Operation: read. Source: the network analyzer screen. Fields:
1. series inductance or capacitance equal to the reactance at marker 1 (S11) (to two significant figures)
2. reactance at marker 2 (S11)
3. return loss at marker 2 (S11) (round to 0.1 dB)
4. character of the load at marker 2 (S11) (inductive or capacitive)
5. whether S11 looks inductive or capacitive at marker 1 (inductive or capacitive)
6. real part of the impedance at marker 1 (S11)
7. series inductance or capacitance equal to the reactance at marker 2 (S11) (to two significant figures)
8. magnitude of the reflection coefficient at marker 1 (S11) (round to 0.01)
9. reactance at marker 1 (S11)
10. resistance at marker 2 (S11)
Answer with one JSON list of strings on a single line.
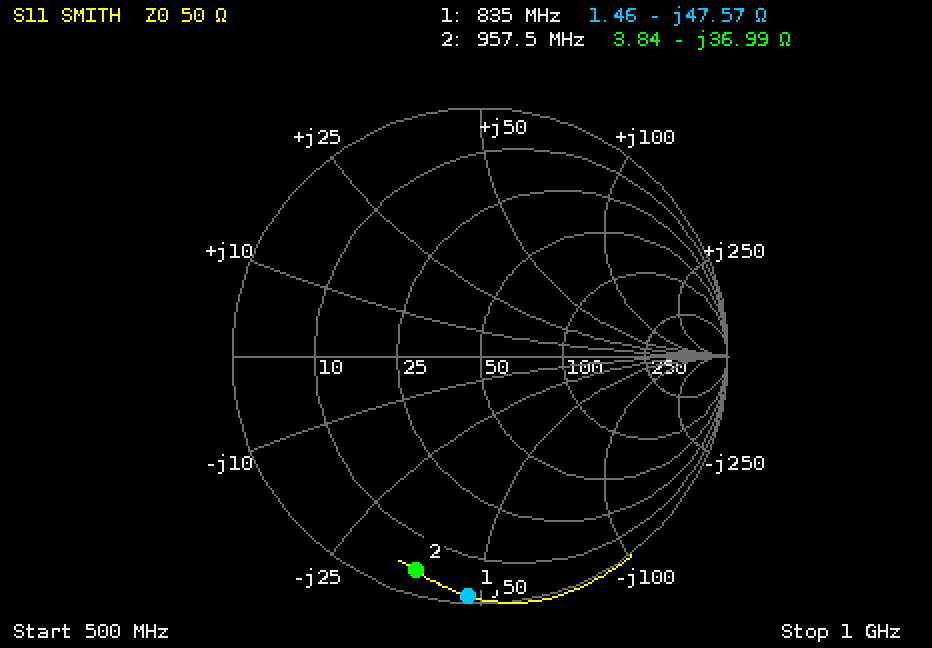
["4.0 pF", "-36.99 Ω", "0.9 dB", "capacitive", "capacitive", "1.46 Ω", "4.5 pF", "0.97", "-47.57 Ω", "3.84 Ω"]
